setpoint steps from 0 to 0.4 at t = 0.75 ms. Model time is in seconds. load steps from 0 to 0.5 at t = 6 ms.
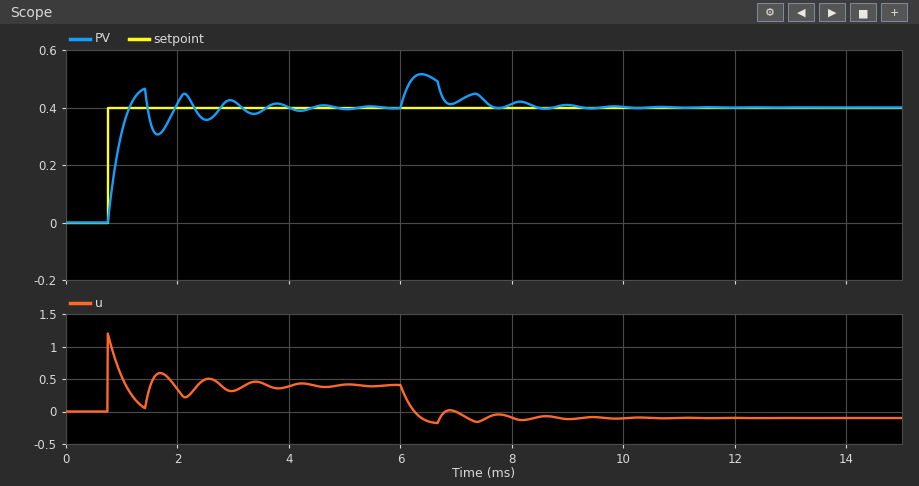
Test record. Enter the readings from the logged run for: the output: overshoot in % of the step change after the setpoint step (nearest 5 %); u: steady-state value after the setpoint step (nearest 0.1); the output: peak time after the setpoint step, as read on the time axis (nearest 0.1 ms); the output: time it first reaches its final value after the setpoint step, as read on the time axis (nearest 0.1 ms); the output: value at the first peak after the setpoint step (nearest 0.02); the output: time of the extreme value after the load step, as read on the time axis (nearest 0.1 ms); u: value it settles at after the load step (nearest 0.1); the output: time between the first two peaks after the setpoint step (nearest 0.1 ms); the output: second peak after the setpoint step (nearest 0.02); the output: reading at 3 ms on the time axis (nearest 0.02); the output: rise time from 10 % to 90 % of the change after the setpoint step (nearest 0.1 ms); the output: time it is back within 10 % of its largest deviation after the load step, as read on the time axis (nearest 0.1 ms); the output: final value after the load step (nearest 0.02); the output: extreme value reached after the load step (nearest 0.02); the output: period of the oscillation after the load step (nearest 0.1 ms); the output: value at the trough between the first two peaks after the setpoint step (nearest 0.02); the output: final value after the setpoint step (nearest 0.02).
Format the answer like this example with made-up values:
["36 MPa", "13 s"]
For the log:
["15 %", "0.4", "1.4 ms", "1.1 ms", "0.46", "6.4 ms", "-0.1", "0.7 ms", "0.44", "0.42", "0.3 ms", "8.3 ms", "0.40", "0.52", "1.0 ms", "0.30", "0.40"]
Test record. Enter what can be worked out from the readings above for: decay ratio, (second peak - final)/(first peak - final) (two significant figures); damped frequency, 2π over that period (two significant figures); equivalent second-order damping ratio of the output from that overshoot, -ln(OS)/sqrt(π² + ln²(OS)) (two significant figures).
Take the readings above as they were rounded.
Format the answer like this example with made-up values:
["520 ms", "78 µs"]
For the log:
["0.67", "9.0 rad/ms", "0.52"]
